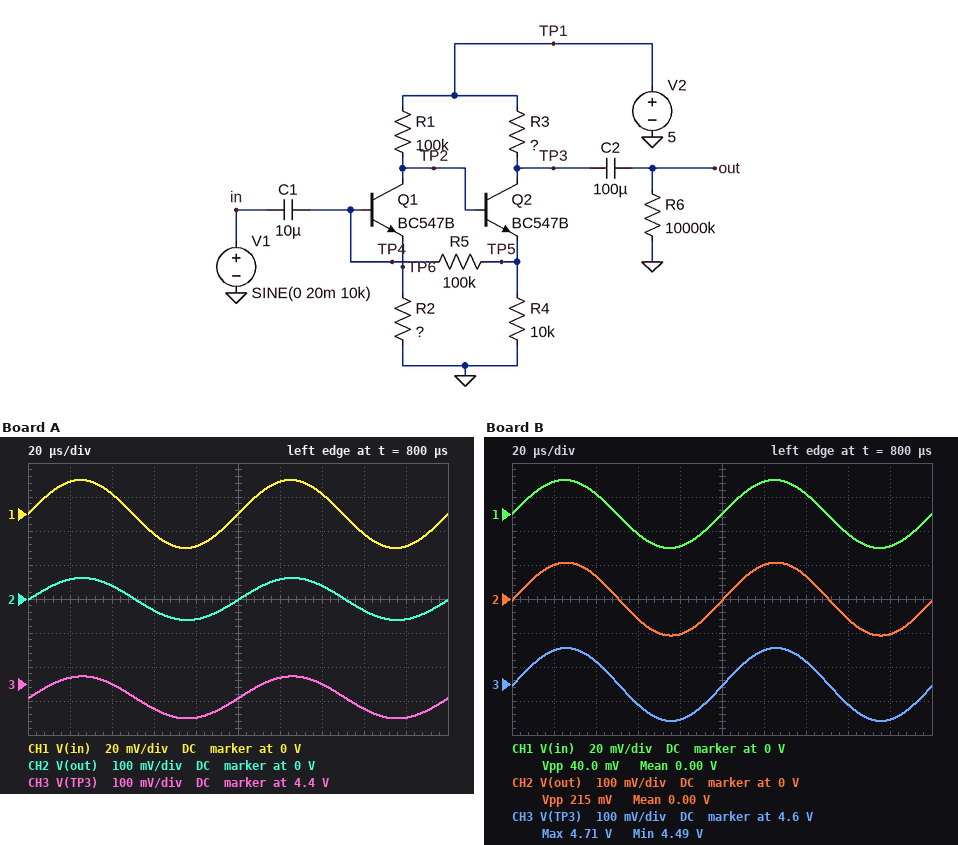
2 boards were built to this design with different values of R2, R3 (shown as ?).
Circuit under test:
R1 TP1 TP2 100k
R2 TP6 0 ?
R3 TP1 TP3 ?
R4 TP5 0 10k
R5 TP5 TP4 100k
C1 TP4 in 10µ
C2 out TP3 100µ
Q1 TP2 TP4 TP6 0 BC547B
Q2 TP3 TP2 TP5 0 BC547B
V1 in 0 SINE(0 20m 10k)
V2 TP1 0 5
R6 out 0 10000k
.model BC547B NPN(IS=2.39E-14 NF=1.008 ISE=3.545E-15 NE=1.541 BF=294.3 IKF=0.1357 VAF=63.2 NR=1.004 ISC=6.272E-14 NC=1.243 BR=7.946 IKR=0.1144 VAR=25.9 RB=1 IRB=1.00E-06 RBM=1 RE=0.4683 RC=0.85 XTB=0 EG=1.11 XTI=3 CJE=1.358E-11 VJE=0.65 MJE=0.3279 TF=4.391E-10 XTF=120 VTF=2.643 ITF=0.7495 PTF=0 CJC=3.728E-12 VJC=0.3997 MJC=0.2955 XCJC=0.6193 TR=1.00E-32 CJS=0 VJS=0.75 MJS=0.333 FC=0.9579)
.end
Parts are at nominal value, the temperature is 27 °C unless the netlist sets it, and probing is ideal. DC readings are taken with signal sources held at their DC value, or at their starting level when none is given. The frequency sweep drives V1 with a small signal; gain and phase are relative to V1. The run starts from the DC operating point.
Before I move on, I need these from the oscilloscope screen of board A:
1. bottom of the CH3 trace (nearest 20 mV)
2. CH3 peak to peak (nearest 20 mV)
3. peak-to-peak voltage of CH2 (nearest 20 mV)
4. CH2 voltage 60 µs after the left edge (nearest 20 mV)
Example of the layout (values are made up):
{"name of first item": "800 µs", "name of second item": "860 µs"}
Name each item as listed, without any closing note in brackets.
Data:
{"bottom of the CH3 trace": "4.30 V", "CH3 peak to peak": "120 mV", "peak-to-peak voltage of CH2": "120 mV", "CH2 voltage 60 µs after the left edge": "-40 mV"}
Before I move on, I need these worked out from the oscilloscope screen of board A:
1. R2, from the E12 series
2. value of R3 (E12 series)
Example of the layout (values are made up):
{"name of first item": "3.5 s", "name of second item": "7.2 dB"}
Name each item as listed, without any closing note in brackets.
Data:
{"R2, from the E12 series": "18 kΩ", "value of R3": "5.6 kΩ"}
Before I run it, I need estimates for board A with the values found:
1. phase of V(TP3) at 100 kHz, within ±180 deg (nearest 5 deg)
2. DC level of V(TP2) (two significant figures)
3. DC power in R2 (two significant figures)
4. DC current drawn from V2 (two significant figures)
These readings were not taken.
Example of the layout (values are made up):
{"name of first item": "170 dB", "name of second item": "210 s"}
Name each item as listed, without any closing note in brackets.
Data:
{"phase of V(TP3) at 100 kHz, within ±180 deg": "-25 deg", "DC level of V(TP2)": "1.7 V", "DC power in R2": "19 µW", "DC current drawn from V2": "150 µA"}
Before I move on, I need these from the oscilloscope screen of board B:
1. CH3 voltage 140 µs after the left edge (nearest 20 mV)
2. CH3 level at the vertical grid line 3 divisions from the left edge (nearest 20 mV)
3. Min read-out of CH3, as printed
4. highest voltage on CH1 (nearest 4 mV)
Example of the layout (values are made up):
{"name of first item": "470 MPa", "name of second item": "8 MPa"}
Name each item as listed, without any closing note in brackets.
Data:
{"CH3 voltage 140 µs after the left edge": "4.66 V", "CH3 level at the vertical grid line 3 divisions from the left edge": "4.54 V", "Min read-out of CH3, as printed": "4.49 V", "highest voltage on CH1": "20 mV"}
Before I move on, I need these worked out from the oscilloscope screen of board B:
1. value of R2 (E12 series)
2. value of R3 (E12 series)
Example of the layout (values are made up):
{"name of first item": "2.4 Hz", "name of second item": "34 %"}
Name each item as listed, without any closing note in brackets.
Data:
{"value of R2": "8.2 kΩ", "value of R3": "4.7 kΩ"}
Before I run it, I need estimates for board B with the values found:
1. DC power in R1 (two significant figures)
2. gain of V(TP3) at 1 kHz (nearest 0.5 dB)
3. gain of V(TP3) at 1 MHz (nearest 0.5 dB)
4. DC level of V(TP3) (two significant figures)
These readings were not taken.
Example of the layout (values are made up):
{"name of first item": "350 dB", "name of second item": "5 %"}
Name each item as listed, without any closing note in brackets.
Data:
{"DC power in R1": "130 µW", "gain of V(TP3) at 1 kHz": "14.5 dB", "gain of V(TP3) at 1 MHz": "2.5 dB", "DC level of V(TP3)": "4.6 V"}
